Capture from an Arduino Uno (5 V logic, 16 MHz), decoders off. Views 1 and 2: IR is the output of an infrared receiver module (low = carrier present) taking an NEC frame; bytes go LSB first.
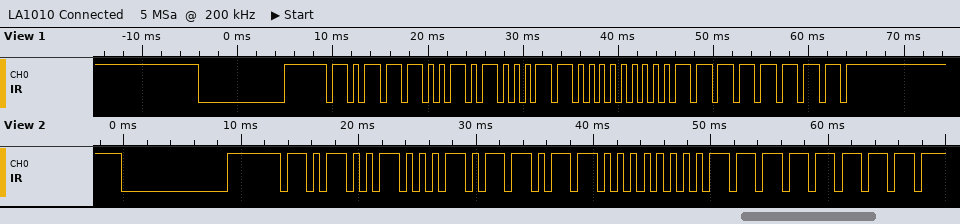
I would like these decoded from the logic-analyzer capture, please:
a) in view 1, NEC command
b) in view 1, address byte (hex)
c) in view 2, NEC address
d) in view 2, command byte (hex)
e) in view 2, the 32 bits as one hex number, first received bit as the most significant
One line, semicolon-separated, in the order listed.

0x00; 0x9D; 0x25; 0x00; 0xA45B00FF
